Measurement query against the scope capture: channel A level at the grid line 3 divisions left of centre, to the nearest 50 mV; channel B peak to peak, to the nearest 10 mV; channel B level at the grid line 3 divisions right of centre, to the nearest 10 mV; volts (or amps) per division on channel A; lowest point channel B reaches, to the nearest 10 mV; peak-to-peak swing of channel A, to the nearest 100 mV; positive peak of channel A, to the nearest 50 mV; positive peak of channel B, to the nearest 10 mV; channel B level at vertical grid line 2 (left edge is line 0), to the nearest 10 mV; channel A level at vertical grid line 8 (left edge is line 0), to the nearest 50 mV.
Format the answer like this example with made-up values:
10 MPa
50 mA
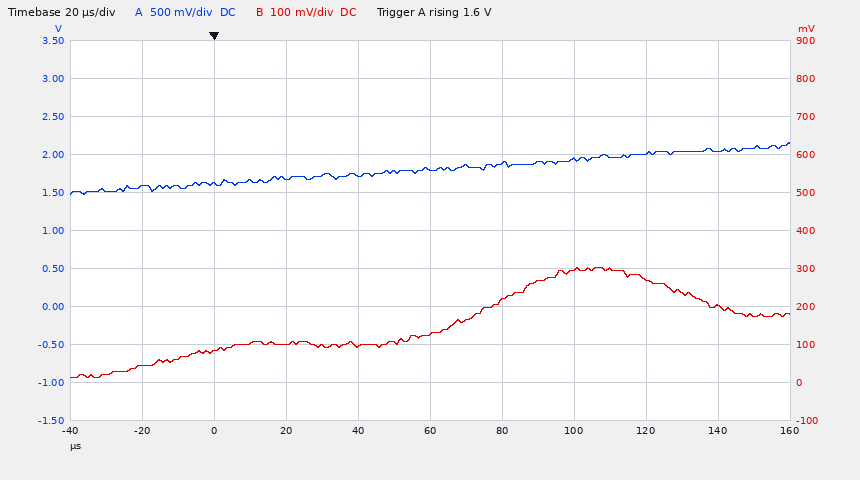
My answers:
1.60 V
290 mV
270 mV
500 mV
10 mV
700 mV
2.15 V
300 mV
80 mV
2.00 V
